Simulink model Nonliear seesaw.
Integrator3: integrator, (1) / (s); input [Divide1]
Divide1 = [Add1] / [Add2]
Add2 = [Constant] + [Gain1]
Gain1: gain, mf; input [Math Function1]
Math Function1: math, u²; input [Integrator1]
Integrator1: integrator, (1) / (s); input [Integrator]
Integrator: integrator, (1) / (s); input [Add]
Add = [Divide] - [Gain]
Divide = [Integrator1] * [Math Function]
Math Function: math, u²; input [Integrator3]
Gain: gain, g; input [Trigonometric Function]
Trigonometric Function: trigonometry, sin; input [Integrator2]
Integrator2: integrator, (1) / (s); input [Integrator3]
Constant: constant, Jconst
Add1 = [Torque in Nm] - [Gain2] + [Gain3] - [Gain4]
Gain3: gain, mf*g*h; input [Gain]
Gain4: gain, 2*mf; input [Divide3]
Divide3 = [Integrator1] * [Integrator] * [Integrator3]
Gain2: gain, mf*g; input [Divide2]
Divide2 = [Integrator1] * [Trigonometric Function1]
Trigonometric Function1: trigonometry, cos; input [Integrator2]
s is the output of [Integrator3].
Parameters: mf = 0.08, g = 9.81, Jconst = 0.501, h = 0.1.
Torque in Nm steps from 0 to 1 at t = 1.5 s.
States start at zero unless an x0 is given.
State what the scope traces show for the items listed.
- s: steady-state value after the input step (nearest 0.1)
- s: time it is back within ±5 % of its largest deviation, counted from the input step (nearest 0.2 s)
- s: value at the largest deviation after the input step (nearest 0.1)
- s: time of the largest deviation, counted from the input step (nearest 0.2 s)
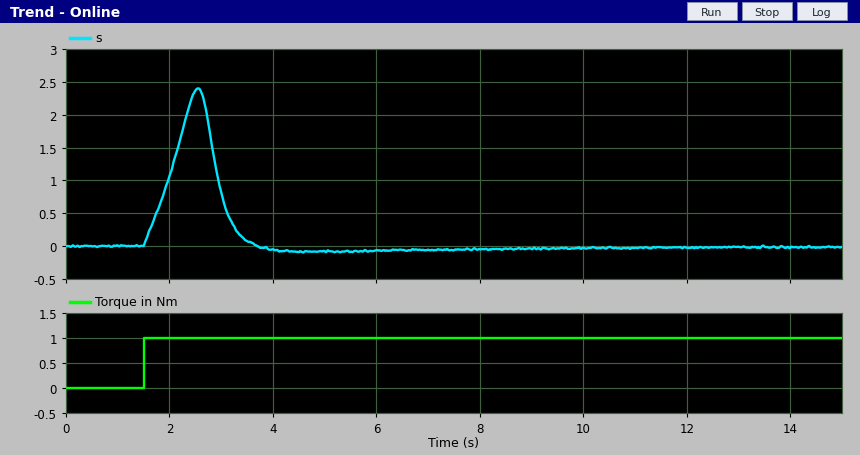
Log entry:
0.0
2.0 s
2.4
1.0 s
